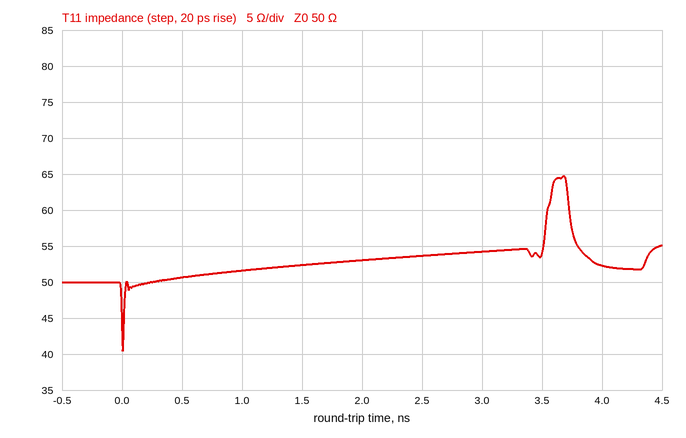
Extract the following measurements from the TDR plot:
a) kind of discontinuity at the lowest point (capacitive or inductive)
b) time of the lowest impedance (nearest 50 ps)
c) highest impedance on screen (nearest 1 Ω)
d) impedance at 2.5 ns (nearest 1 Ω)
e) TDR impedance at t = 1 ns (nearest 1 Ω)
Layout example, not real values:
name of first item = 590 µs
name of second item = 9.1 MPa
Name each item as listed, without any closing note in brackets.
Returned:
kind of discontinuity at the lowest point = capacitive
time of the lowest impedance = 0 ps
highest impedance on screen = 65 Ω
impedance at 2.5 ns = 54 Ω
TDR impedance at t = 1 ns = 52 Ω
